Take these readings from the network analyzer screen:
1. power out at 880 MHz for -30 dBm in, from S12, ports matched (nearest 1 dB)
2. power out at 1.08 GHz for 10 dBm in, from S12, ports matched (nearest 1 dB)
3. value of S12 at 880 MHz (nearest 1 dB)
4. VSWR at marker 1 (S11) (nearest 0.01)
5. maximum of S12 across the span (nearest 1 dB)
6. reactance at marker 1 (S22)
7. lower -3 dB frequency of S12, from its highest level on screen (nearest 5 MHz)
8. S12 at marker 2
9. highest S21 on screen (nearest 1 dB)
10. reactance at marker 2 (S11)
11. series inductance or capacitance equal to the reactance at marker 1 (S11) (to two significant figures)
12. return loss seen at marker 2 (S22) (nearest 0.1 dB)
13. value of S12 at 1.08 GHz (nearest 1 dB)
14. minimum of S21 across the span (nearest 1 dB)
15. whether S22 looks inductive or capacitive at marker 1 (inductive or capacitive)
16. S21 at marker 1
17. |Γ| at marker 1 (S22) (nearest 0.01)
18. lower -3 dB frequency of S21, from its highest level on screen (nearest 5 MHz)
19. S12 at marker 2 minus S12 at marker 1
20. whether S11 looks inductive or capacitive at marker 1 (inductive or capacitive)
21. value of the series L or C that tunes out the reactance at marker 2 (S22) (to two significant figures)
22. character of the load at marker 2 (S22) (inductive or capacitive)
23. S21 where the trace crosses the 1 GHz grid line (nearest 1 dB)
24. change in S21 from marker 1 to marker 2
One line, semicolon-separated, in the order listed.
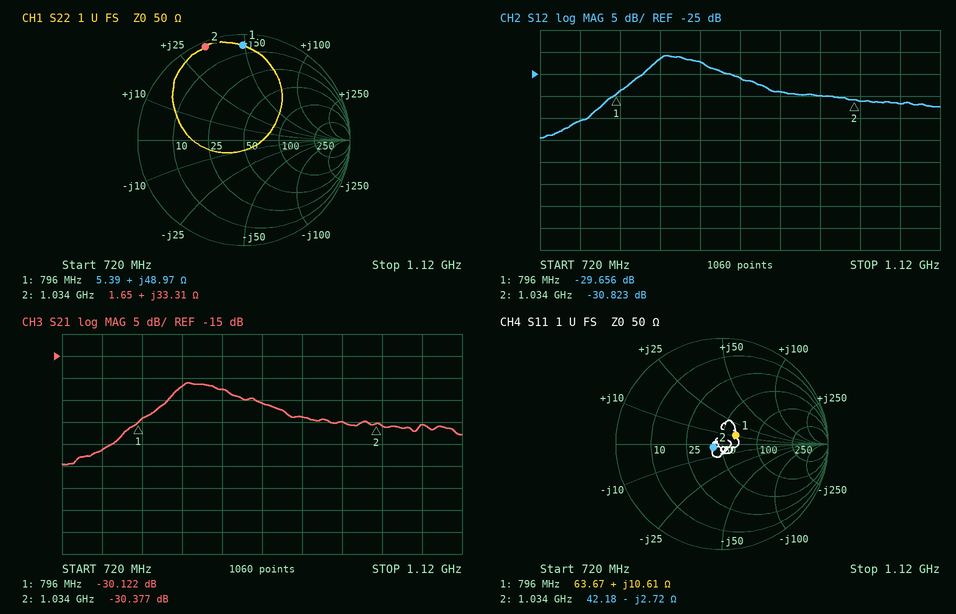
-52 dBm; -22 dBm; -22 dB; 1.36; -21 dB; +48.97 Ω; 830 MHz; -30.823 dB; -21 dB; -2.72 Ω; 2.1 nH; 0.4 dB; -32 dB; -40 dB; inductive; -30.122 dB; 0.90; 830 MHz; -1.167 dB; inductive; 4.6 pF; inductive; -30 dB; -0.255 dB
